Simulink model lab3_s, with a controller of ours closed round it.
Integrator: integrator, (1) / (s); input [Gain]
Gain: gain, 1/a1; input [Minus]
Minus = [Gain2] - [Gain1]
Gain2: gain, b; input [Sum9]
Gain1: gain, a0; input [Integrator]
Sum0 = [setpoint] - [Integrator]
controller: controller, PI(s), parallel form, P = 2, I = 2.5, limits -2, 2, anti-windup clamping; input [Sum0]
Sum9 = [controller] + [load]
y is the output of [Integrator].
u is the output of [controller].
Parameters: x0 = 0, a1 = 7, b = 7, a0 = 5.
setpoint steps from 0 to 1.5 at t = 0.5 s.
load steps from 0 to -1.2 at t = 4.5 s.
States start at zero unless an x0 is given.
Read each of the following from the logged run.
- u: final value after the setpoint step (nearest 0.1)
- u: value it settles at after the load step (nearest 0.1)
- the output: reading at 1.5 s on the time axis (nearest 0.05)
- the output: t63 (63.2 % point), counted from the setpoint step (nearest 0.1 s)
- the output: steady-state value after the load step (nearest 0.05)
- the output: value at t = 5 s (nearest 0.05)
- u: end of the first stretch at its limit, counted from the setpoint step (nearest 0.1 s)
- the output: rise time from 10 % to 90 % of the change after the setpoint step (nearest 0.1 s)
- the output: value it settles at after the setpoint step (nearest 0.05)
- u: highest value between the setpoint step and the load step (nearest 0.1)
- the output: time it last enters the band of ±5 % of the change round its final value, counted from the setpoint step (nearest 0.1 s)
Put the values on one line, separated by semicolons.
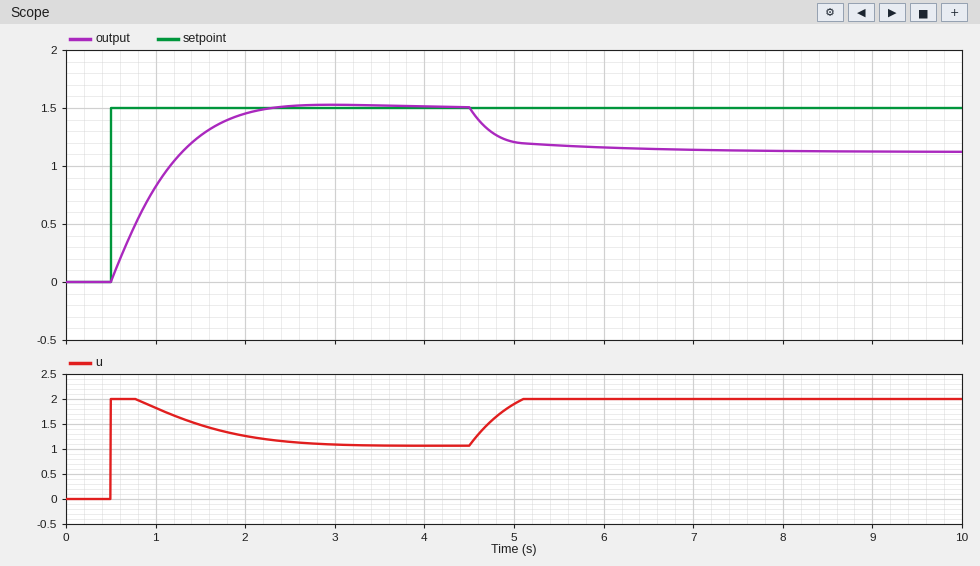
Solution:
1.1; 2.0; 1.25; 0.6 s; 1.10; 1.20; 0.3 s; 1.1 s; 1.50; 2.0; 1.4 s
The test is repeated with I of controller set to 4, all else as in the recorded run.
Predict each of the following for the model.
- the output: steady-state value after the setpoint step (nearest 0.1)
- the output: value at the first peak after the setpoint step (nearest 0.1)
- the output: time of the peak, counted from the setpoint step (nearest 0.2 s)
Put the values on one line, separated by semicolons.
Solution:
1.5; 1.6; 1.8 s
